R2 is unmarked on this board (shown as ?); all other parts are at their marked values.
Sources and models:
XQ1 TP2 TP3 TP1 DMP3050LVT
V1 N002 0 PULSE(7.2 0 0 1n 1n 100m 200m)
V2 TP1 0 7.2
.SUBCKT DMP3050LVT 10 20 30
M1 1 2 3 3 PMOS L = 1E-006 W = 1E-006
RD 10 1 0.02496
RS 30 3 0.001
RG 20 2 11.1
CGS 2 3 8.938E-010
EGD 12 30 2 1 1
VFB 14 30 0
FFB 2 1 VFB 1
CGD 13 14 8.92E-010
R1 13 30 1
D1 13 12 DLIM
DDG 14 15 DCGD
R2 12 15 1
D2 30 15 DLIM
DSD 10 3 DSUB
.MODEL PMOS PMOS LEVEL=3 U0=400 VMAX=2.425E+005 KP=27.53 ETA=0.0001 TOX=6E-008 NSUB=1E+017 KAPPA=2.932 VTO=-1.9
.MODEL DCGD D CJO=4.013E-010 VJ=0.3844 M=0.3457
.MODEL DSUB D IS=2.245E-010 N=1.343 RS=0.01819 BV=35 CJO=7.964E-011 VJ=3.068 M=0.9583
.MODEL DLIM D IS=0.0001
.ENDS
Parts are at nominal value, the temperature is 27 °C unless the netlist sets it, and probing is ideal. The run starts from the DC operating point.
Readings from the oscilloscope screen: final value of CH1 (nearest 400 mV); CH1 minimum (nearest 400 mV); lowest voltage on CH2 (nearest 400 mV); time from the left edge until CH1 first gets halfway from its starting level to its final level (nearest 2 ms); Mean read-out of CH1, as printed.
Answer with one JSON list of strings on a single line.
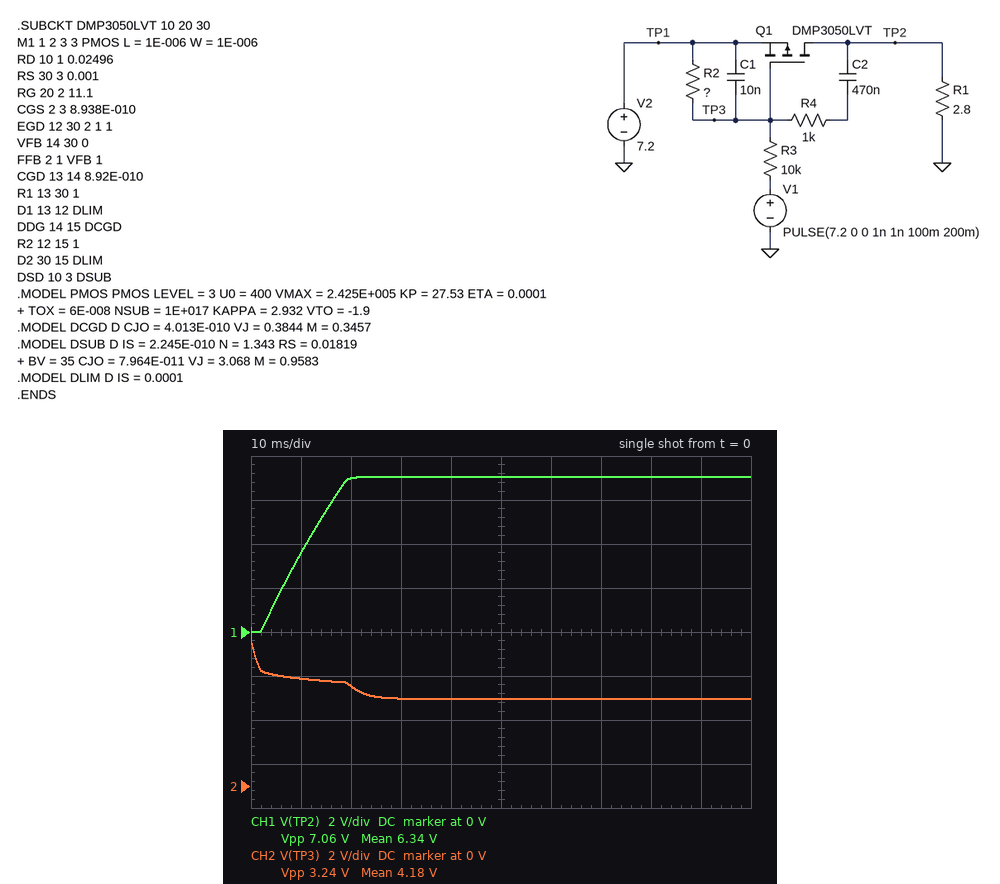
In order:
["7.2 V", "0 V", "4.0 V", "10 ms", "6.34 V"]
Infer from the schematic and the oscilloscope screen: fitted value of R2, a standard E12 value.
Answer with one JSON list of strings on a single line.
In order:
["8.2 kΩ"]
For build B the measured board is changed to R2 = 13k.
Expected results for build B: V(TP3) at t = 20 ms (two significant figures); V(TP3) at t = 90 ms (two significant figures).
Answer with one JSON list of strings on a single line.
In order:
["3.3 V", "3.1 V"]
